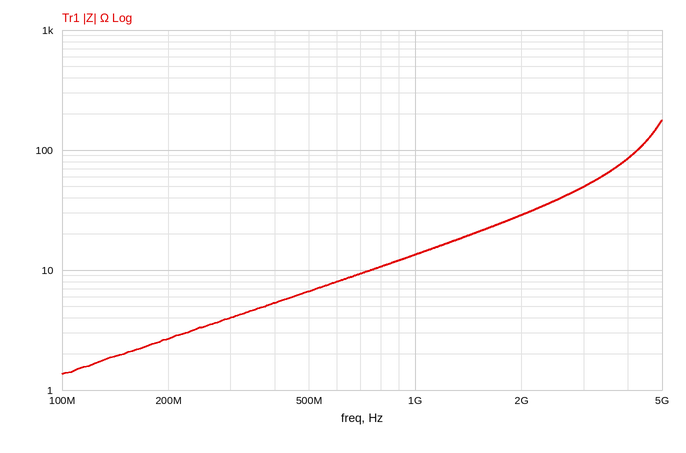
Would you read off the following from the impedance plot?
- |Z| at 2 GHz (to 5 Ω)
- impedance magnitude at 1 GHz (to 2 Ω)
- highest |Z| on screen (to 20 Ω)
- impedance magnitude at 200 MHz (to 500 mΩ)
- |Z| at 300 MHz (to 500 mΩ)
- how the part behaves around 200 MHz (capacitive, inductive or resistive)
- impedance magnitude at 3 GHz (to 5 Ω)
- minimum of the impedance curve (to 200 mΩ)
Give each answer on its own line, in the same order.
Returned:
30 Ω
14 Ω
180 Ω
2.5 Ω
4.0 Ω
inductive
50 Ω
1.4 Ω
